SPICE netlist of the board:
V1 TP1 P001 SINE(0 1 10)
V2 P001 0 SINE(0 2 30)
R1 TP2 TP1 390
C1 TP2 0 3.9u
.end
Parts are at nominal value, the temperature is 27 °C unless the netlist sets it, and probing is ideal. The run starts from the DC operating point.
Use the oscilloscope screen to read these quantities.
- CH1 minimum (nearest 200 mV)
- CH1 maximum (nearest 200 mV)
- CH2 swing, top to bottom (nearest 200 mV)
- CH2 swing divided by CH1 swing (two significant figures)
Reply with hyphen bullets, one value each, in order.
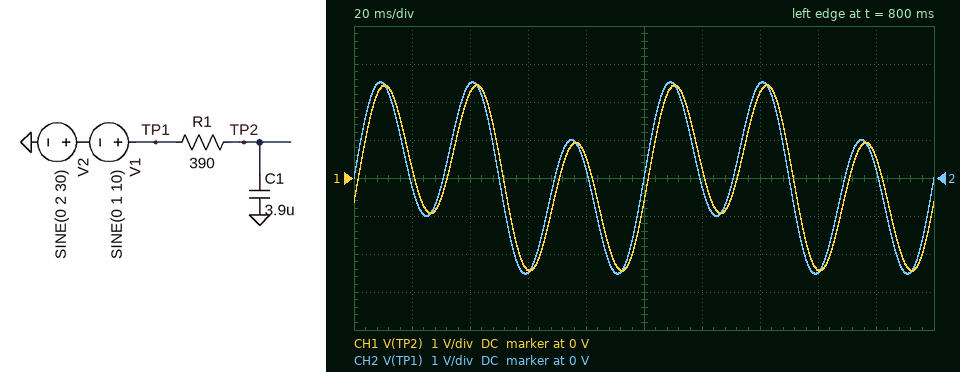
- -2.4 V
- 2.4 V
- 5.0 V
- 1.0
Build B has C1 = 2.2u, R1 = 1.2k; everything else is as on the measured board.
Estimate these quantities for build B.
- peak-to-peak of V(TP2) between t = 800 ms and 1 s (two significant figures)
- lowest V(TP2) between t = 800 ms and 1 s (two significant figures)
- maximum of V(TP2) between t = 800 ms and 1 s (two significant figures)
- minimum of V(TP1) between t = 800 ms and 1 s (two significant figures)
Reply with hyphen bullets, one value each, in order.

- 4.6 V
- -2.3 V
- 2.3 V
- -2.5 V
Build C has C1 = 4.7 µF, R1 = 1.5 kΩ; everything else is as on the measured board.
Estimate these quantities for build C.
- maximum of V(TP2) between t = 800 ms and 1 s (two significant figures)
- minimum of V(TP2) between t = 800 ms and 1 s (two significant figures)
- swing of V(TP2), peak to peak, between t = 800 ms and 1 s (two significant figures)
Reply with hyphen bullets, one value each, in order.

- 1.8 V
- -1.8 V
- 3.5 V
